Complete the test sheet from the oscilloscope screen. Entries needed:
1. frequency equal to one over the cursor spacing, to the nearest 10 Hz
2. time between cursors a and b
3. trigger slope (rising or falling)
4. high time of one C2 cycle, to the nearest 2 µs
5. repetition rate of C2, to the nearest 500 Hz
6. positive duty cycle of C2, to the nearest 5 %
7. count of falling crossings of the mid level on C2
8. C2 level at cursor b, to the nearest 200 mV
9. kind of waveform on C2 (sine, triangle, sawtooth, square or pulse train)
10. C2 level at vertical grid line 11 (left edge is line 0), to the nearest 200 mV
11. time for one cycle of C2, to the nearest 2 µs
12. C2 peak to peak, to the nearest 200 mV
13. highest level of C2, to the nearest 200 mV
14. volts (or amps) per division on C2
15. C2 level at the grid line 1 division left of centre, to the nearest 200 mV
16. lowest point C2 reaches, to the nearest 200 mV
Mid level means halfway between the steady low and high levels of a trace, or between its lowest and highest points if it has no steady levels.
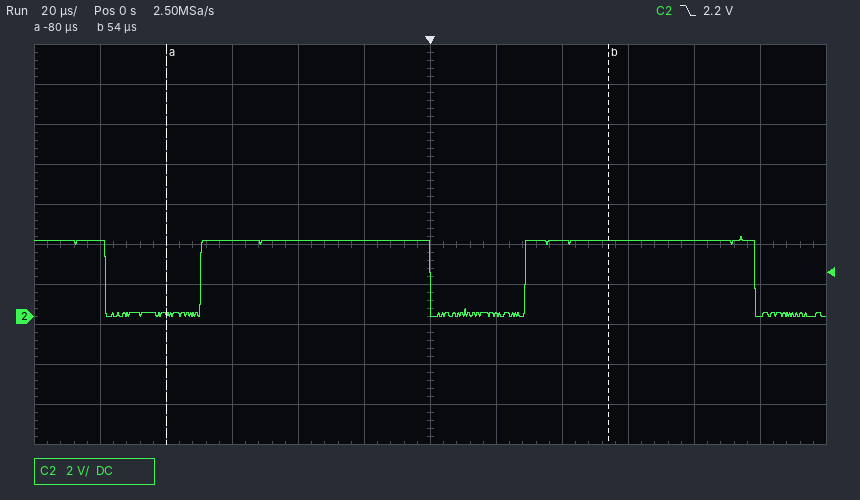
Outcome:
7.46 kHz
134 µs
falling
70 µs
10.0 kHz
70 %
3
3.8 V
pulse train
0.0 V
98 µs
4.0 V
4.0 V
2 V
3.8 V
0.0 V
